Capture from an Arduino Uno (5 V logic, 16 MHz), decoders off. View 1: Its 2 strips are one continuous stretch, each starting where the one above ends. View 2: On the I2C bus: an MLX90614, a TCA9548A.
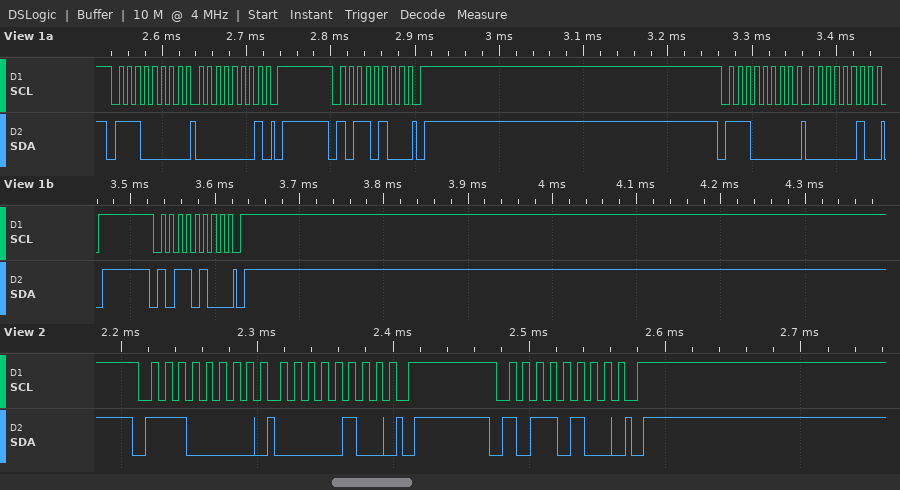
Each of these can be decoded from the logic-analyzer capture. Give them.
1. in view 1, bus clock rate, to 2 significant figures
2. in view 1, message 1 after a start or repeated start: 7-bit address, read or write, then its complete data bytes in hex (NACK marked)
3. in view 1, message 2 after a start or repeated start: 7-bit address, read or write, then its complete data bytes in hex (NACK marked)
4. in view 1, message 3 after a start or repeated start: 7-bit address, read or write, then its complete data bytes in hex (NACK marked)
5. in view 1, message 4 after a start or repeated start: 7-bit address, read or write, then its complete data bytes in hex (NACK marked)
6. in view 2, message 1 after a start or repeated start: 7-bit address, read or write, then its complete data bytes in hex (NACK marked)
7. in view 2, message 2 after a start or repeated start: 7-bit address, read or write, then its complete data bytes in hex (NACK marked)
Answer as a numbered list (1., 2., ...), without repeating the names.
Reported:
1. 100 kHz
2. 0x70 write: 01
3. 0x5A write
4. 0x70 write: 02
5. 0x5A write
6. 0x70 write: 04
7. 0x5A write
